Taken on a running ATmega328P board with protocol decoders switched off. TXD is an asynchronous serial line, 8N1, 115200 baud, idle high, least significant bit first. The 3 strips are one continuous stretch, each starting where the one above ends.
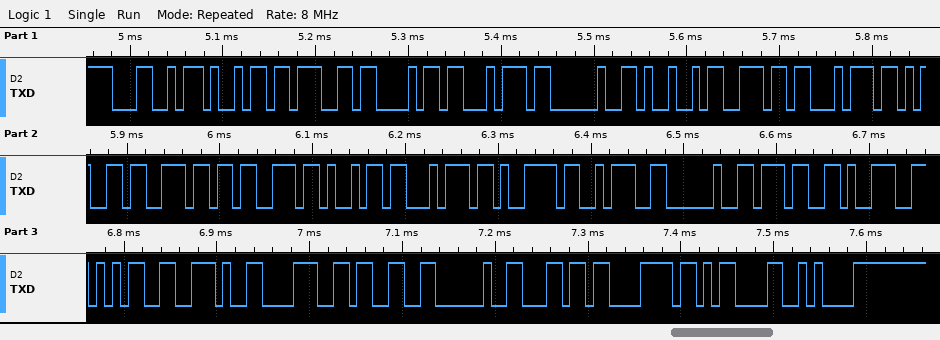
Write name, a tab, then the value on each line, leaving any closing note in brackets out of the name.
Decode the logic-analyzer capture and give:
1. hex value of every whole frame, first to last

hex value of every whole frame, first to last	4C 69 67 68 74 20 49 6E 74 65 6E 73 69 74 79 3A 20 37 39 35 2E 38 33 20 6C 78 0D 0A
